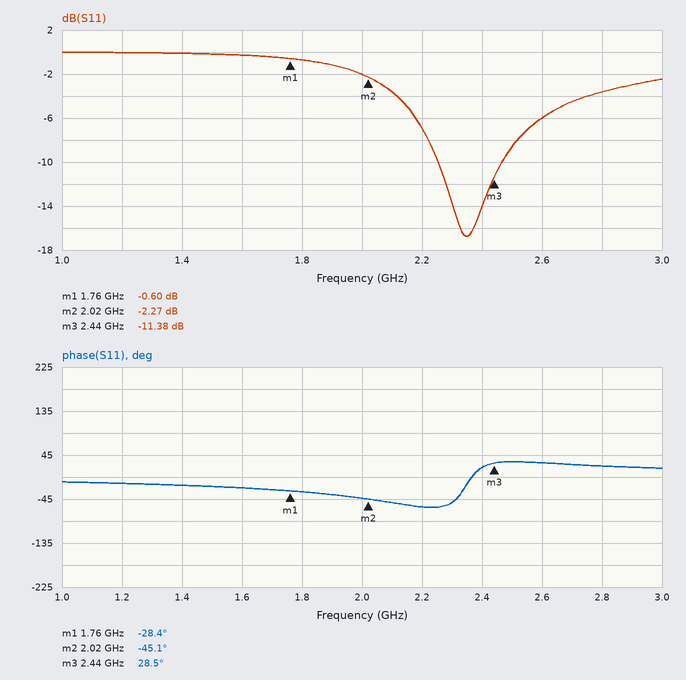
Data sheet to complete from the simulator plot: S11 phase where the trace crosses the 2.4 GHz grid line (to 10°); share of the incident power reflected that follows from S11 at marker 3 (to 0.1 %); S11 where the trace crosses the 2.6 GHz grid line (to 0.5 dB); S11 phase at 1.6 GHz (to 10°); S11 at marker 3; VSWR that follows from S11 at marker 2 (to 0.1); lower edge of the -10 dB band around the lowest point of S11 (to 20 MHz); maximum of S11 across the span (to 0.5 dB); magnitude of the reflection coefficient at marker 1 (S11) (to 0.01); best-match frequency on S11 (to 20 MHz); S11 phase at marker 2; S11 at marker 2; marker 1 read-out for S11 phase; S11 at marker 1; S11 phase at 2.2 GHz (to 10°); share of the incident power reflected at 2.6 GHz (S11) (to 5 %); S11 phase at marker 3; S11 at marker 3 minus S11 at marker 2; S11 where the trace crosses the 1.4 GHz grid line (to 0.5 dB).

20°
7.3 %
-6.0 dB
-20°
-11.38 dB
7.7
2.26 GHz
0.0 dB
0.93
2.34 GHz
-45.1°
-2.27 dB
-28.4°
-0.60 dB
-60°
25 %
28.5°
-9.11 dB
0.0 dB
